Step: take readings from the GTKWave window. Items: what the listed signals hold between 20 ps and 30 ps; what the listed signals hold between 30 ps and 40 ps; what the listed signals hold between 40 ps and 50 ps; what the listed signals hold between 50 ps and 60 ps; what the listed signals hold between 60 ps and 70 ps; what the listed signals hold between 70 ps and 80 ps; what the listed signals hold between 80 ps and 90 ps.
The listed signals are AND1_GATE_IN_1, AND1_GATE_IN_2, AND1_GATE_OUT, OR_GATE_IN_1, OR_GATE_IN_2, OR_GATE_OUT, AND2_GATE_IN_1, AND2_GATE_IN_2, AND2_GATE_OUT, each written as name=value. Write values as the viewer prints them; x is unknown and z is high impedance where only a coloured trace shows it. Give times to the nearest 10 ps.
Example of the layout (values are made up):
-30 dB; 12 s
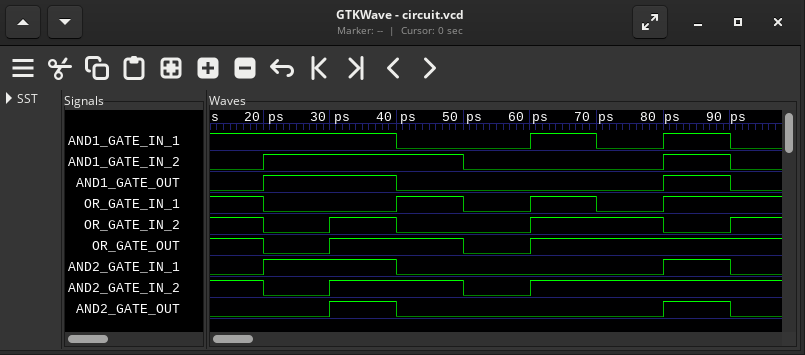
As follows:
AND1_GATE_IN_1=1, AND1_GATE_IN_2=1, AND1_GATE_OUT=1, OR_GATE_IN_1=0, OR_GATE_IN_2=0, OR_GATE_OUT=0, AND2_GATE_IN_1=1, AND2_GATE_IN_2=0, AND2_GATE_OUT=0; AND1_GATE_IN_1=1, AND1_GATE_IN_2=1, AND1_GATE_OUT=1, OR_GATE_IN_1=0, OR_GATE_IN_2=1, OR_GATE_OUT=1, AND2_GATE_IN_1=1, AND2_GATE_IN_2=1, AND2_GATE_OUT=1; AND1_GATE_IN_1=0, AND1_GATE_IN_2=1, AND1_GATE_OUT=0, OR_GATE_IN_1=1, OR_GATE_IN_2=0, OR_GATE_OUT=1, AND2_GATE_IN_1=0, AND2_GATE_IN_2=1, AND2_GATE_OUT=0; AND1_GATE_IN_1=0, AND1_GATE_IN_2=0, AND1_GATE_OUT=0, OR_GATE_IN_1=0, OR_GATE_IN_2=0, OR_GATE_OUT=0, AND2_GATE_IN_1=0, AND2_GATE_IN_2=0, AND2_GATE_OUT=0; AND1_GATE_IN_1=1, AND1_GATE_IN_2=0, AND1_GATE_OUT=0, OR_GATE_IN_1=1, OR_GATE_IN_2=1, OR_GATE_OUT=1, AND2_GATE_IN_1=0, AND2_GATE_IN_2=1, AND2_GATE_OUT=0; AND1_GATE_IN_1=0, AND1_GATE_IN_2=0, AND1_GATE_OUT=0, OR_GATE_IN_1=0, OR_GATE_IN_2=1, OR_GATE_OUT=1, AND2_GATE_IN_1=0, AND2_GATE_IN_2=1, AND2_GATE_OUT=0; AND1_GATE_IN_1=1, AND1_GATE_IN_2=1, AND1_GATE_OUT=1, OR_GATE_IN_1=1, OR_GATE_IN_2=0, OR_GATE_OUT=1, AND2_GATE_IN_1=1, AND2_GATE_IN_2=1, AND2_GATE_OUT=1
